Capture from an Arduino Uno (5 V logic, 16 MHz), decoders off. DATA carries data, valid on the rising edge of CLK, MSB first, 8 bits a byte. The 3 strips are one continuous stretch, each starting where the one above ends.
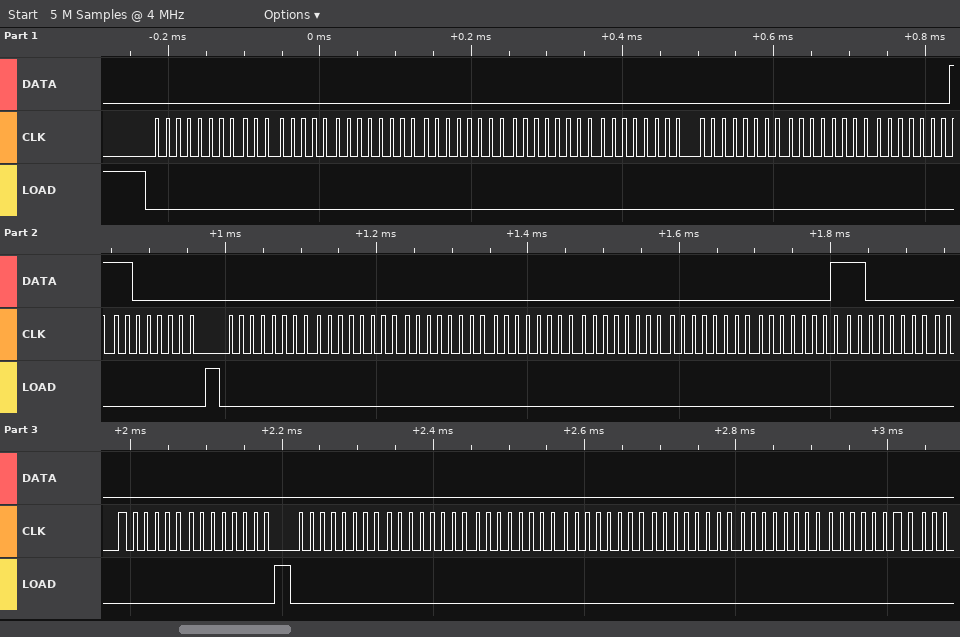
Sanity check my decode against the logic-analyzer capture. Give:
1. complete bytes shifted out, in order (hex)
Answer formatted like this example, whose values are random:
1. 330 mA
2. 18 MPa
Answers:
1. 0x00 0x00 0x00 0x00 0x00 0x00 0x00 0x00 0x01 0xC0 0x00 0x00 0x00 0x00 0x00 0x00 0x01 0xC0 0x00 0x00 0x00 0x00 0x00 0x00 0x00 0x00 0x00
